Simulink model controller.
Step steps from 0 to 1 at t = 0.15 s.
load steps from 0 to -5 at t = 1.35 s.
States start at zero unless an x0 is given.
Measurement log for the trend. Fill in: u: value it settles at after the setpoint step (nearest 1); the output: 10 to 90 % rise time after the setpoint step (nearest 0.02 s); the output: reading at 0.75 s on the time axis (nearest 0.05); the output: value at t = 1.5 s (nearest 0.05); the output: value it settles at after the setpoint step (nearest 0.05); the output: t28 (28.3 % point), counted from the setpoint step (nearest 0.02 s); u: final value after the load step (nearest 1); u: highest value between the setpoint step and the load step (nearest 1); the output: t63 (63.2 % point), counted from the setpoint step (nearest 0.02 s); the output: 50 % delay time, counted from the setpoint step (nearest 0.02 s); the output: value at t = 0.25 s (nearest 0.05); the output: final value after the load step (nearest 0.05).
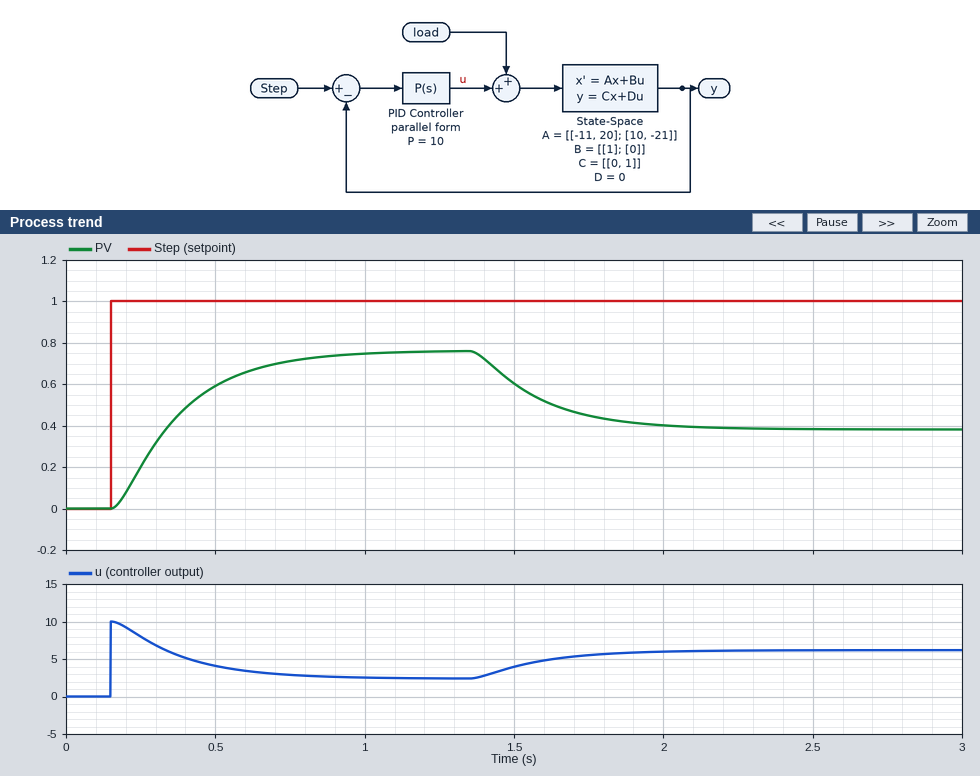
2
0.46 s
0.70
0.60
0.75
0.10 s
6
10
0.24 s
0.18 s
0.20
0.40
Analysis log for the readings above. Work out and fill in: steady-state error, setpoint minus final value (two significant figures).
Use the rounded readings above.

0.25
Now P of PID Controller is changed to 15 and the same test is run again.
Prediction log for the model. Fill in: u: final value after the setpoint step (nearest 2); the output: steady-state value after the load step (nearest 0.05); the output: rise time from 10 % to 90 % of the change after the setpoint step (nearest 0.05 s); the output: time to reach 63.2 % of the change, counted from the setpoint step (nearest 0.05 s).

2
0.55
0.30 s
0.20 s
